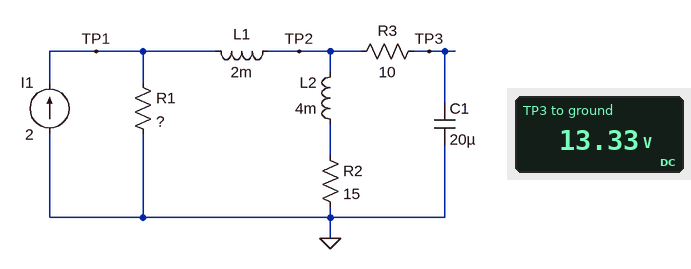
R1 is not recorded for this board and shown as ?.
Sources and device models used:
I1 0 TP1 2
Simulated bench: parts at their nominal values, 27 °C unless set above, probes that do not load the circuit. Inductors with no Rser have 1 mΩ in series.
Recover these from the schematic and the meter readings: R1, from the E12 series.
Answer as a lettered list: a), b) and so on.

a) 12 Ω
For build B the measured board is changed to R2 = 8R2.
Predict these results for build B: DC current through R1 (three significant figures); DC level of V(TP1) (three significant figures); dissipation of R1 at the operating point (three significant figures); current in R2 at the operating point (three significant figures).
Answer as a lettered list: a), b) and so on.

a) 812 mA
b) 9.74 V
c) 7.91 W
d) 1.19 A
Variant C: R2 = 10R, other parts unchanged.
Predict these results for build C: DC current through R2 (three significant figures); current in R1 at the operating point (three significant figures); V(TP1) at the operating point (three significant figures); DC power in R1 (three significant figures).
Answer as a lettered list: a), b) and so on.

a) 1.09 A
b) 909 mA
c) 10.9 V
d) 9.92 W
